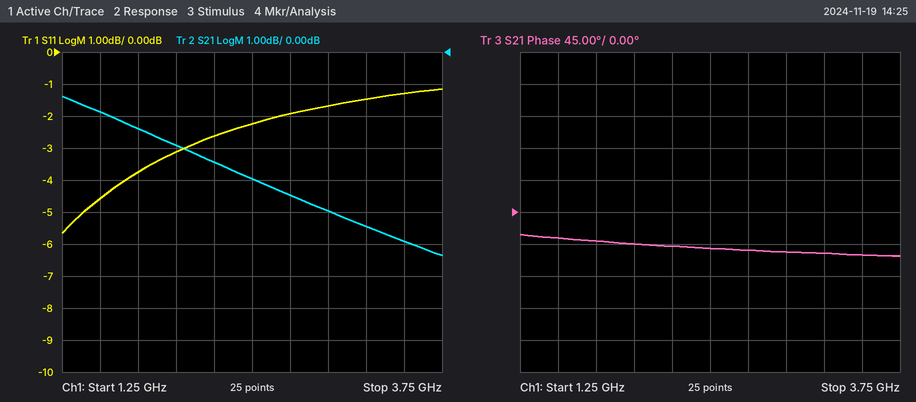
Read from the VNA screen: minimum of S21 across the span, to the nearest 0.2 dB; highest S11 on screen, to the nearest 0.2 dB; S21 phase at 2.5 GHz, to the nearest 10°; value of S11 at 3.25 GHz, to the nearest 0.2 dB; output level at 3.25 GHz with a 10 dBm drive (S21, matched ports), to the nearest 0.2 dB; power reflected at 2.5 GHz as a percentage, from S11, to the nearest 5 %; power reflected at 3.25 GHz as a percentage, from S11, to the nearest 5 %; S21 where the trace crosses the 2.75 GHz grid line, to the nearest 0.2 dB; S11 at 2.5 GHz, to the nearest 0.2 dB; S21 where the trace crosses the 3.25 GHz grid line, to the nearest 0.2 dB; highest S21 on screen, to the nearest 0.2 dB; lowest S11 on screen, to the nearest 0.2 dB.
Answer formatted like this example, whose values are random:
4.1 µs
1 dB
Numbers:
-6.4 dB
-1.2 dB
-50°
-1.4 dB
4.6 dBm
60 %
70 %
-4.4 dB
-2.2 dB
-5.4 dB
-1.4 dB
-5.6 dB
